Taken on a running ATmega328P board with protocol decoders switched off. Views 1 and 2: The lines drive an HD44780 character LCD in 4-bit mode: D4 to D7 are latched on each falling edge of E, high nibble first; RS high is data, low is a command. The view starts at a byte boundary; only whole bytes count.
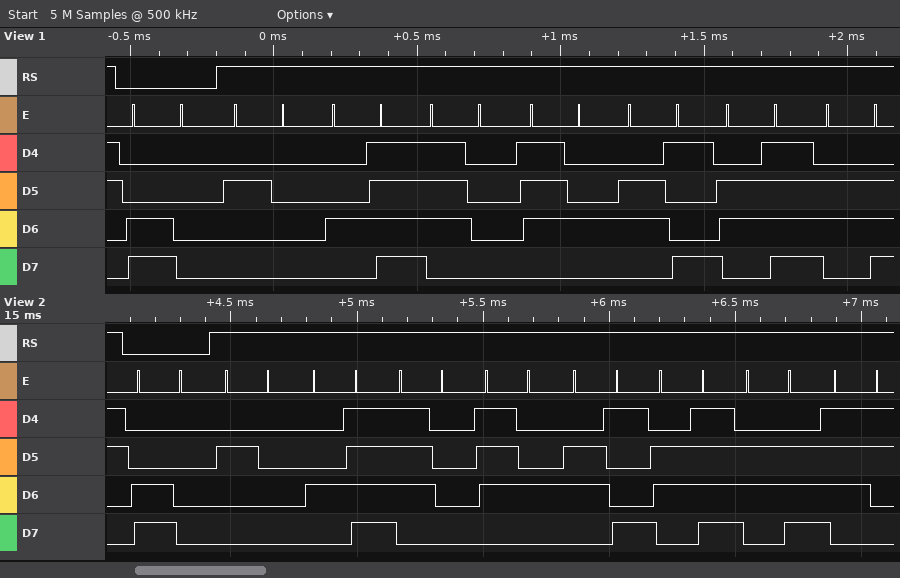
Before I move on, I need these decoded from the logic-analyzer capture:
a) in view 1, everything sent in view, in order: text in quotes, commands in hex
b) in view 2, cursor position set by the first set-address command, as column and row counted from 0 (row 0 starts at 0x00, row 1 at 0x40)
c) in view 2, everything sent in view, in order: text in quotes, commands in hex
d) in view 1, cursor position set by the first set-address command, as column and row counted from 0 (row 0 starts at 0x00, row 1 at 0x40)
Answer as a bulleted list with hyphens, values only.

- 0xC0 " Option"
- column 0, row 1
- 0xC0 " Options"
- column 0, row 1
